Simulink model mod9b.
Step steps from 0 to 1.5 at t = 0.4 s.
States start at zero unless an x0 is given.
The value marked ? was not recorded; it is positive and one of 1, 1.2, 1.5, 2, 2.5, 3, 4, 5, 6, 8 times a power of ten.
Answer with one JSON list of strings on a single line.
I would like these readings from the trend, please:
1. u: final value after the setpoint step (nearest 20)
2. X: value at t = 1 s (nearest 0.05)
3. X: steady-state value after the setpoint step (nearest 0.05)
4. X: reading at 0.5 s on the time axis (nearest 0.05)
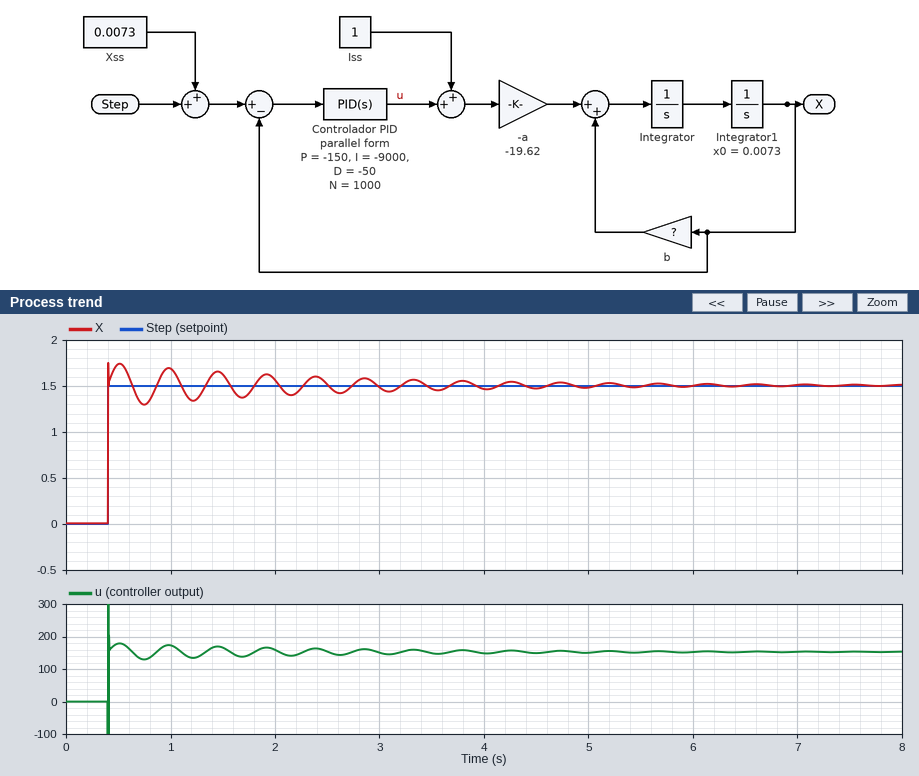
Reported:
["160", "1.70", "1.50", "1.75"]
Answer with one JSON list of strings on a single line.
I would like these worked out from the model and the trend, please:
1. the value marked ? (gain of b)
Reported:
["2000"]
